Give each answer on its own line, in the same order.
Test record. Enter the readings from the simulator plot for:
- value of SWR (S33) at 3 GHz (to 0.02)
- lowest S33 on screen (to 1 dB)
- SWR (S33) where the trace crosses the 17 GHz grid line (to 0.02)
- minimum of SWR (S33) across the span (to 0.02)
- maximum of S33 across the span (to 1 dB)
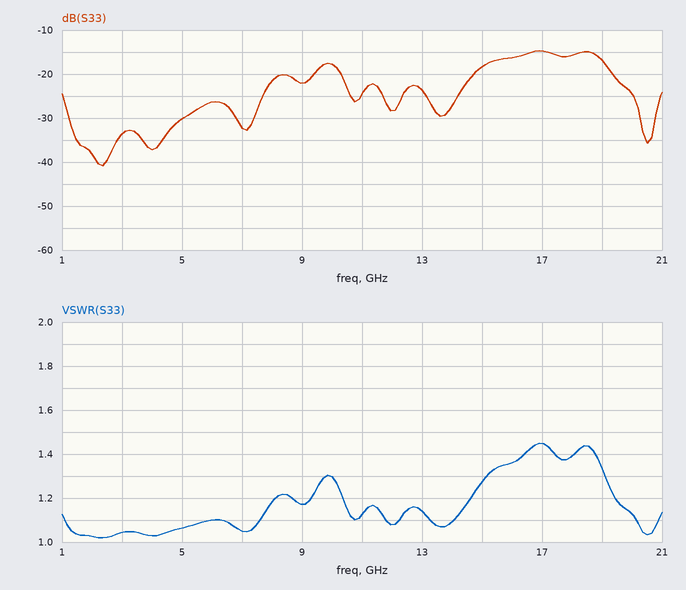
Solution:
1.04
-41 dB
1.44
1.02
-15 dB
